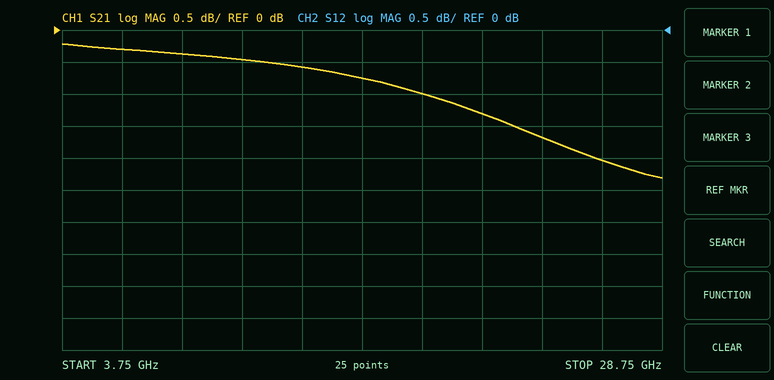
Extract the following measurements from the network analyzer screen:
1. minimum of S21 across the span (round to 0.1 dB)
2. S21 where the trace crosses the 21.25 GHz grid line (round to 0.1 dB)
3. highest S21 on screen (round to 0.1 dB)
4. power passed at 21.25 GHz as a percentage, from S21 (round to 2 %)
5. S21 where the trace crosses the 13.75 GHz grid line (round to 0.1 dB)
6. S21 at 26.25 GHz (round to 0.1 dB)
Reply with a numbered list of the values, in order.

1. -2.3 dB
2. -1.3 dB
3. -0.2 dB
4. 74 %
5. -0.6 dB
6. -2.0 dB
